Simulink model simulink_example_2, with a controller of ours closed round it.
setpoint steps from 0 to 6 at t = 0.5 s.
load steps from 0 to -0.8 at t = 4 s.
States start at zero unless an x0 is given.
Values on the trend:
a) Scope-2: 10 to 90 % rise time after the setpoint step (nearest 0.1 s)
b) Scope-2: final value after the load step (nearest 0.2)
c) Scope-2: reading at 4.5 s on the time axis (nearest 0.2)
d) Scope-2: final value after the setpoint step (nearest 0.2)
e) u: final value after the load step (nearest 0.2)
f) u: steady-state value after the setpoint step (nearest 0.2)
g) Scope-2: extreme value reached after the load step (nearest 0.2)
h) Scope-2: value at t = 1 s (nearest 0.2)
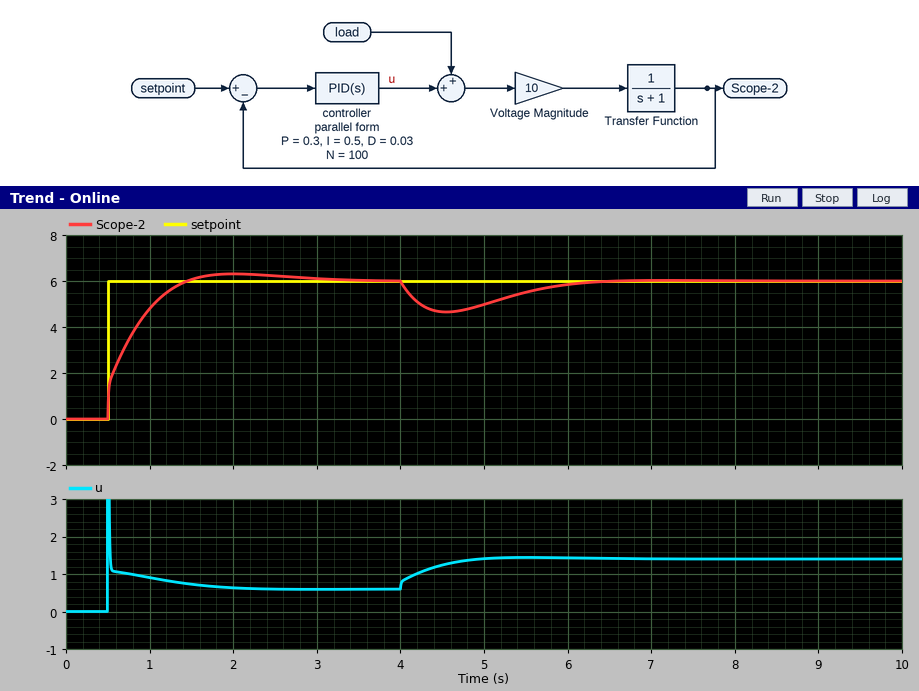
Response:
0.7 s
6.0
4.6
6.0
1.4
0.6
4.6
4.8
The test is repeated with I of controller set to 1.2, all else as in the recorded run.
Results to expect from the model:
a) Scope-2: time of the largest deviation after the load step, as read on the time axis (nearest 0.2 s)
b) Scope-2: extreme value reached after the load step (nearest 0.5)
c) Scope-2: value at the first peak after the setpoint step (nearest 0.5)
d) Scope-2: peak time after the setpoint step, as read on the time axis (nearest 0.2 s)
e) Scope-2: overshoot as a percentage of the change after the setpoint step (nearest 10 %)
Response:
4.4 s
5.0
7.0
1.4 s
20 %
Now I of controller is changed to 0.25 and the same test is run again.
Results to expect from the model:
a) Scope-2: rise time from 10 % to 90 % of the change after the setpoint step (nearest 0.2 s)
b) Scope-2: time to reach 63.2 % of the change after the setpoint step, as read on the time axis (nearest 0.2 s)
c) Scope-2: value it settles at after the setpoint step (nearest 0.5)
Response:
1.0 s
0.8 s
6.0
